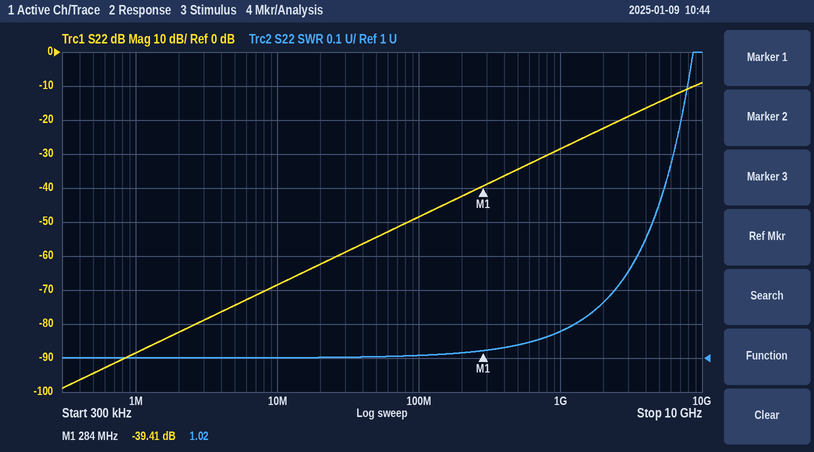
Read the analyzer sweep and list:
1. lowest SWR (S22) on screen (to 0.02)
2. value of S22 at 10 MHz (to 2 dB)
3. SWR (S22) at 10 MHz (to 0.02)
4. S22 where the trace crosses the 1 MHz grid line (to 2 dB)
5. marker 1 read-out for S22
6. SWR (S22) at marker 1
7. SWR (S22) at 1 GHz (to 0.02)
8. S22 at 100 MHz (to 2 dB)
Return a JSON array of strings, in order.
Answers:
["1.00", "-68 dB", "1.00", "-88 dB", "-39.41 dB", "1.02", "1.08", "-48 dB"]
